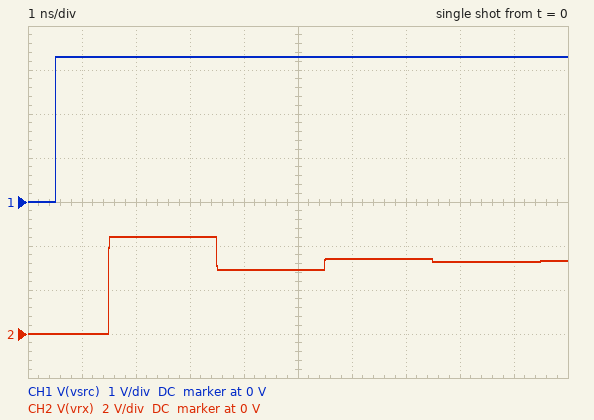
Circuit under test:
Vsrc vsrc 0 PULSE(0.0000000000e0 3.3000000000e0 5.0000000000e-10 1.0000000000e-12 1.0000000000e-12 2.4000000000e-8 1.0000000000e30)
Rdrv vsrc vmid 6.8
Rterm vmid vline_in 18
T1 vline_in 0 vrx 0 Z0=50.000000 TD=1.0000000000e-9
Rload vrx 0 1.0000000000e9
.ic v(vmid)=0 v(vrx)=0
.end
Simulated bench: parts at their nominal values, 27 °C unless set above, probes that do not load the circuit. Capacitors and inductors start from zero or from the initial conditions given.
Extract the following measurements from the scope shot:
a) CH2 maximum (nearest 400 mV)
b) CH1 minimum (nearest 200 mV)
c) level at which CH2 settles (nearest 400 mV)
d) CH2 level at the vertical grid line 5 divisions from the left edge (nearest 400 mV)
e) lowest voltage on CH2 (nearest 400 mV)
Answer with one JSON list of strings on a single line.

["4.4 V", "0 V", "3.2 V", "2.8 V", "0 V"]
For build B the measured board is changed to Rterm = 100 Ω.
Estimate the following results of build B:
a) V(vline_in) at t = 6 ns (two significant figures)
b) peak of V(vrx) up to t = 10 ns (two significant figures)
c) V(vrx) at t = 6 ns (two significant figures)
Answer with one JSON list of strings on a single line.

["3.0 V", "3.3 V", "3.1 V"]
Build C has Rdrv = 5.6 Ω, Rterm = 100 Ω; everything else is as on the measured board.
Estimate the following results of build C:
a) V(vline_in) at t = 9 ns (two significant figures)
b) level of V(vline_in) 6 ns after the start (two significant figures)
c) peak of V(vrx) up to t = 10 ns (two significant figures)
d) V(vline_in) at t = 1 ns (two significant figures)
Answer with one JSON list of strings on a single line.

["3.3 V", "3.0 V", "3.3 V", "1.1 V"]
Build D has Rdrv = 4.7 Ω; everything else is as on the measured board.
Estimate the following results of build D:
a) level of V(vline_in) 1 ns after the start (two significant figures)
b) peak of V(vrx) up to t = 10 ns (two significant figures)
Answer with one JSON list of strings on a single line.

["2.3 V", "4.5 V"]
